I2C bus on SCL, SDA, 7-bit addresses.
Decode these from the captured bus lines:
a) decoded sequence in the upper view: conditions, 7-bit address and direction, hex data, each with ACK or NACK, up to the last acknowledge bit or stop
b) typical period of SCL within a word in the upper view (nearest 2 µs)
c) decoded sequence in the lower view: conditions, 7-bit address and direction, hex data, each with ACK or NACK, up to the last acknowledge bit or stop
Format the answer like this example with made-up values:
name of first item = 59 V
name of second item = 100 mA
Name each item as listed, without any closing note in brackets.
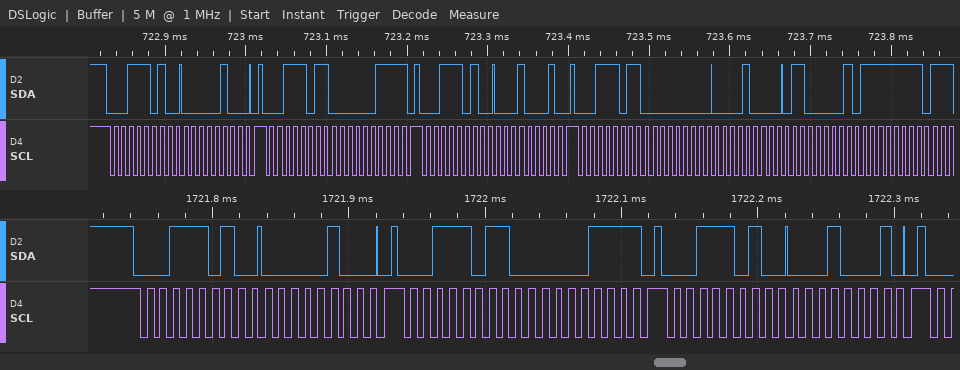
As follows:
decoded sequence in the upper view: conditions, 7-bit address and direction, hex data, each with ACK or NACK, up to the last acknowledge bit or stop = start, address 1D write ACK, 04 ACK, stop, start, address 1D read ACK, 07 NACK, stop, start, address 1D write ACK, 11 ACK, stop, start, address 1D read ACK, 00 ACK, 10 ACK, C1 ACK, FF ACK
typical period of SCL within a word in the upper view = 10 µs
decoded sequence in the lower view: conditions, 7-bit address and direction, hex data, each with ACK or NACK, up to the last acknowledge bit or stop = start, address 1D write ACK, 04 ACK, stop, start, address 1D read ACK, 07 NACK, stop, start, address 1D write ACK, 11 ACK, stop
